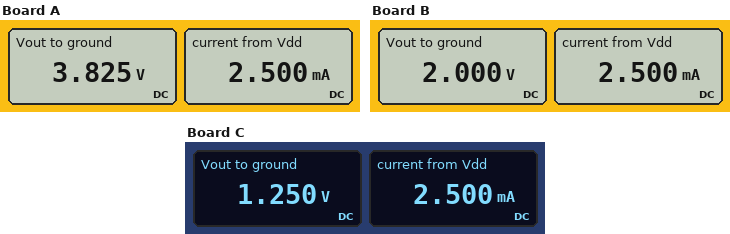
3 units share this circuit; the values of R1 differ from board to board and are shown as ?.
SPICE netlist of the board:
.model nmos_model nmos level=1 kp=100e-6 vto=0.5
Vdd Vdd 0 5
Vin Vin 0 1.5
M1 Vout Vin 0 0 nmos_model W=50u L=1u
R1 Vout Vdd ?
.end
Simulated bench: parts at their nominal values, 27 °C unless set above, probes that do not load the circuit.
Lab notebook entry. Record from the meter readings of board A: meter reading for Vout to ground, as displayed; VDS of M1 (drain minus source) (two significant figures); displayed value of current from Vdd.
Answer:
3.825 V
3.8 V
2.500 mA
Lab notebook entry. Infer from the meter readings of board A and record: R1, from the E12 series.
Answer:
470 Ω
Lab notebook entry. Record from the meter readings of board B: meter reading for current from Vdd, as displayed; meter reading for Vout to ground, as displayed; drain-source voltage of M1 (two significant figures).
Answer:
2.500 mA
2.000 V
2.0 V
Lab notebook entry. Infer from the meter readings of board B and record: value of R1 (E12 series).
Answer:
1.2 kΩ
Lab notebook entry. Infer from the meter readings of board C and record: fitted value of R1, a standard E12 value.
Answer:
1.5 kΩ
